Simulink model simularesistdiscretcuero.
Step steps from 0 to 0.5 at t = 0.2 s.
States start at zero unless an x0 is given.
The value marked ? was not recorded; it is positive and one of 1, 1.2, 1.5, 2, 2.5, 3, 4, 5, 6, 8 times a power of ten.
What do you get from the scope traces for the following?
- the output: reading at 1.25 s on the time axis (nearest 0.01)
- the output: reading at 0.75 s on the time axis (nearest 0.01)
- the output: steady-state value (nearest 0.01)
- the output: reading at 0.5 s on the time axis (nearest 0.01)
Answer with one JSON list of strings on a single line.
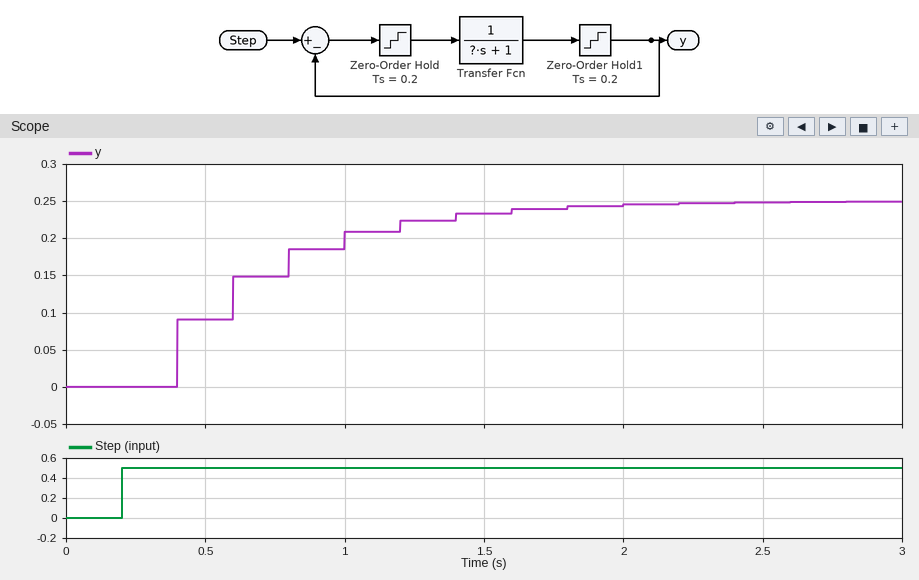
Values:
["0.22", "0.15", "0.25", "0.09"]
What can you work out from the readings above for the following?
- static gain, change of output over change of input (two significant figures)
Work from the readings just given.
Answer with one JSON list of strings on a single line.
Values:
["0.50"]
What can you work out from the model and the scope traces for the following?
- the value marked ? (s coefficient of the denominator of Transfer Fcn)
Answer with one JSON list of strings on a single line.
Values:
["1"]
